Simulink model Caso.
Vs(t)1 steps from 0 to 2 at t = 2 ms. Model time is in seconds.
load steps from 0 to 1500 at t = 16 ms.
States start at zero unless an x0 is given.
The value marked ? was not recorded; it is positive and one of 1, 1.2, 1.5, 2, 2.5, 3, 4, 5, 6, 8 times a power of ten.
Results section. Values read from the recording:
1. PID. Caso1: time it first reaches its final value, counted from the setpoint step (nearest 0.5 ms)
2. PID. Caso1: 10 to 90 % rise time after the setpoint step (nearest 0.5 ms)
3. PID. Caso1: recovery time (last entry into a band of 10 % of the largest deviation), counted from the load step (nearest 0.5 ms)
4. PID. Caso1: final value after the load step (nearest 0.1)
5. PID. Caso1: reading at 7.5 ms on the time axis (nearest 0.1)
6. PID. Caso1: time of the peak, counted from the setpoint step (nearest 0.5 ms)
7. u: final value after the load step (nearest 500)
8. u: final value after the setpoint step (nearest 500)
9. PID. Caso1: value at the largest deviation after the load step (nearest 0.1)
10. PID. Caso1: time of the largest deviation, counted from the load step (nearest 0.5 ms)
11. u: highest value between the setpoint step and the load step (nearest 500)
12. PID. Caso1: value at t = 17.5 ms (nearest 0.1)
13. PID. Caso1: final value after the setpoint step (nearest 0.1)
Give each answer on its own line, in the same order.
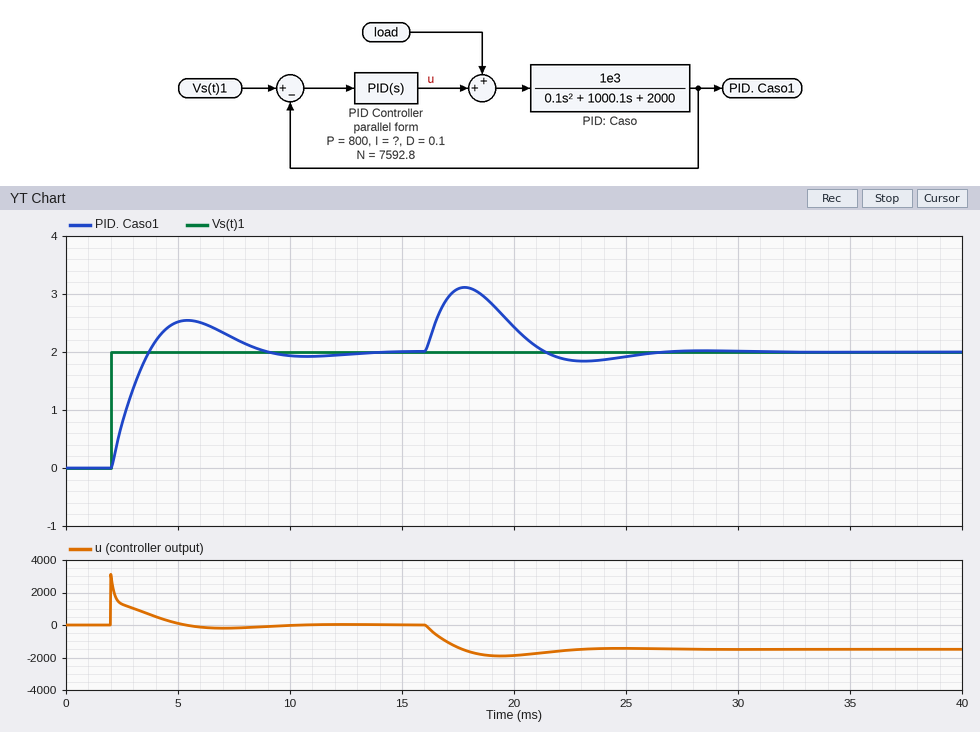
1.5 ms
1.5 ms
8.5 ms
2.0
2.2
3.5 ms
-1500
0
3.1
2.0 ms
3000
3.1
2.0
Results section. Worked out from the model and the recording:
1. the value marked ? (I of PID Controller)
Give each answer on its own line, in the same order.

500000
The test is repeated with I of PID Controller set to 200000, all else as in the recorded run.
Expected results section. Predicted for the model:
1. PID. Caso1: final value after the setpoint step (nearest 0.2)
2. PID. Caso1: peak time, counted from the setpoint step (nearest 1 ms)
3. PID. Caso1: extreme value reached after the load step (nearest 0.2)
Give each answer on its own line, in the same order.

2.0
5 ms
3.4
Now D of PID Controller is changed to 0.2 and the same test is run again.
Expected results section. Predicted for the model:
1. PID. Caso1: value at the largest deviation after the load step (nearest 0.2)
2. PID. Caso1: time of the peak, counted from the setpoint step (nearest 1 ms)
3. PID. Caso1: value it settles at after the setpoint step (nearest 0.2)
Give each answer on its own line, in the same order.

3.0
4 ms
2.0
